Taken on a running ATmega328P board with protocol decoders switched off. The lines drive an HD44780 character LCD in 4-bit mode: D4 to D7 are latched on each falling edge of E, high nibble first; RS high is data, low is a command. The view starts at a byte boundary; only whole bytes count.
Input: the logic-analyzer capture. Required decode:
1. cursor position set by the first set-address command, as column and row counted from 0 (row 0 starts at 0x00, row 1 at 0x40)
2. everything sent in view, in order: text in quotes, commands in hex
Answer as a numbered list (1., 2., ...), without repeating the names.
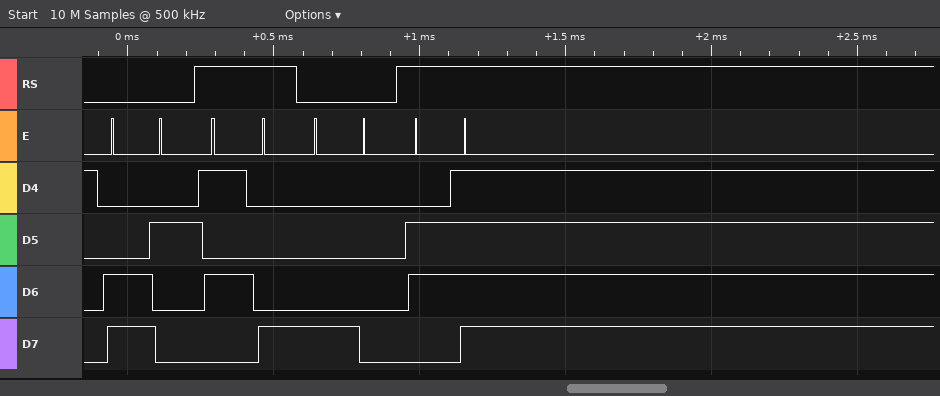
1. column 2, row 1
2. 0xC2 "X" 0x80 "o"
